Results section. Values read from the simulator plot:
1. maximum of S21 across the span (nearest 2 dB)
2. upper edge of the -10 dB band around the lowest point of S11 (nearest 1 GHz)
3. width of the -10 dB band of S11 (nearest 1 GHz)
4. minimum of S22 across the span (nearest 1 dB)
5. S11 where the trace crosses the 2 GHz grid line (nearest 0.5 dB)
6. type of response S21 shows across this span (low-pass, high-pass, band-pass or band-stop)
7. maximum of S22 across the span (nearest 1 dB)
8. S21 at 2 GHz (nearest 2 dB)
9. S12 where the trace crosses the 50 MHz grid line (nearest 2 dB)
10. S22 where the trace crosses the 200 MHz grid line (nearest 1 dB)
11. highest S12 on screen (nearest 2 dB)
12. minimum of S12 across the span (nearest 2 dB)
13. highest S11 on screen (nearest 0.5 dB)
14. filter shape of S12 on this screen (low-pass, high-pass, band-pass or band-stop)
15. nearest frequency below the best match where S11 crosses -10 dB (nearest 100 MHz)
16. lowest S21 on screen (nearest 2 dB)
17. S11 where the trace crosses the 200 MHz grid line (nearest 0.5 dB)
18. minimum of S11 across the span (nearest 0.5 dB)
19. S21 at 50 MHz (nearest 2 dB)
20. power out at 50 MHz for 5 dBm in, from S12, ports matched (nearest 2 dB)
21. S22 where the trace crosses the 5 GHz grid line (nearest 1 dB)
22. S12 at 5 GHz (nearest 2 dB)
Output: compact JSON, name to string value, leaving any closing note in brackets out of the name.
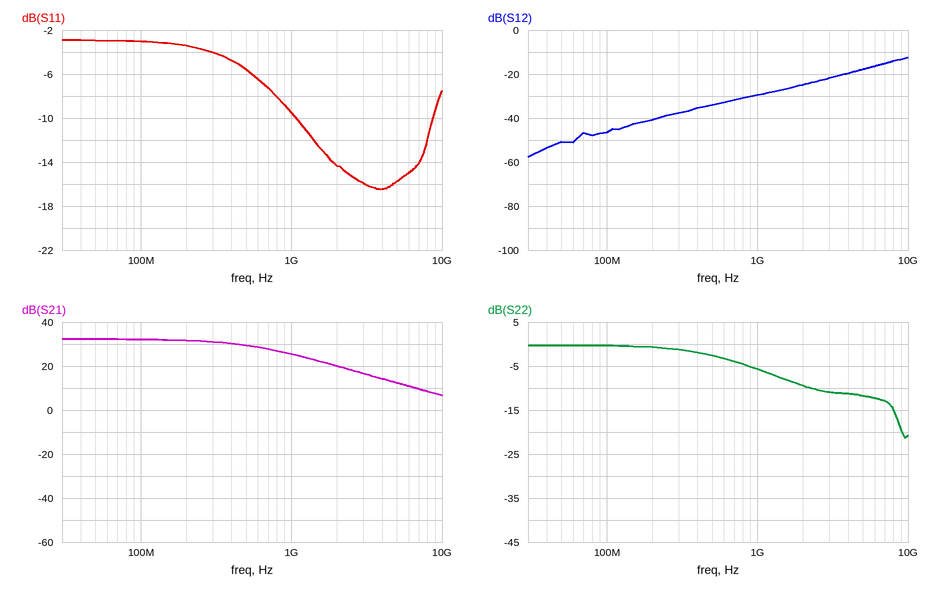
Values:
{"maximum of S21 across the span": "32 dB", "upper edge of the -10 dB band around the lowest point of S11": "9 GHz", "width of the -10 dB band of S11": "8 GHz", "minimum of S22 across the span": "-21 dB", "S11 where the trace crosses the 2 GHz grid line": "-14.5 dB", "type of response S21 shows across this span": "low-pass", "maximum of S22 across the span": "0 dB", "S21 at 2 GHz": "20 dB", "S12 where the trace crosses the 50 MHz grid line": "-50 dB", "S22 where the trace crosses the 200 MHz grid line": "-1 dB", "highest S12 on screen": "-12 dB", "minimum of S12 across the span": "-58 dB", "highest S11 on screen": "-3.0 dB", "filter shape of S12 on this screen": "high-pass", "nearest frequency below the best match where S11 crosses -10 dB": "1.1 GHz", "lowest S21 on screen": "6 dB", "S11 where the trace crosses the 200 MHz grid line": "-3.5 dB", "minimum of S11 across the span": "-16.5 dB", "S21 at 50 MHz": "32 dB", "power out at 50 MHz for 5 dBm in, from S12, ports matched": "-46 dBm", "S22 where the trace crosses the 5 GHz grid line": "-12 dB", "S12 at 5 GHz": "-18 dB"}
